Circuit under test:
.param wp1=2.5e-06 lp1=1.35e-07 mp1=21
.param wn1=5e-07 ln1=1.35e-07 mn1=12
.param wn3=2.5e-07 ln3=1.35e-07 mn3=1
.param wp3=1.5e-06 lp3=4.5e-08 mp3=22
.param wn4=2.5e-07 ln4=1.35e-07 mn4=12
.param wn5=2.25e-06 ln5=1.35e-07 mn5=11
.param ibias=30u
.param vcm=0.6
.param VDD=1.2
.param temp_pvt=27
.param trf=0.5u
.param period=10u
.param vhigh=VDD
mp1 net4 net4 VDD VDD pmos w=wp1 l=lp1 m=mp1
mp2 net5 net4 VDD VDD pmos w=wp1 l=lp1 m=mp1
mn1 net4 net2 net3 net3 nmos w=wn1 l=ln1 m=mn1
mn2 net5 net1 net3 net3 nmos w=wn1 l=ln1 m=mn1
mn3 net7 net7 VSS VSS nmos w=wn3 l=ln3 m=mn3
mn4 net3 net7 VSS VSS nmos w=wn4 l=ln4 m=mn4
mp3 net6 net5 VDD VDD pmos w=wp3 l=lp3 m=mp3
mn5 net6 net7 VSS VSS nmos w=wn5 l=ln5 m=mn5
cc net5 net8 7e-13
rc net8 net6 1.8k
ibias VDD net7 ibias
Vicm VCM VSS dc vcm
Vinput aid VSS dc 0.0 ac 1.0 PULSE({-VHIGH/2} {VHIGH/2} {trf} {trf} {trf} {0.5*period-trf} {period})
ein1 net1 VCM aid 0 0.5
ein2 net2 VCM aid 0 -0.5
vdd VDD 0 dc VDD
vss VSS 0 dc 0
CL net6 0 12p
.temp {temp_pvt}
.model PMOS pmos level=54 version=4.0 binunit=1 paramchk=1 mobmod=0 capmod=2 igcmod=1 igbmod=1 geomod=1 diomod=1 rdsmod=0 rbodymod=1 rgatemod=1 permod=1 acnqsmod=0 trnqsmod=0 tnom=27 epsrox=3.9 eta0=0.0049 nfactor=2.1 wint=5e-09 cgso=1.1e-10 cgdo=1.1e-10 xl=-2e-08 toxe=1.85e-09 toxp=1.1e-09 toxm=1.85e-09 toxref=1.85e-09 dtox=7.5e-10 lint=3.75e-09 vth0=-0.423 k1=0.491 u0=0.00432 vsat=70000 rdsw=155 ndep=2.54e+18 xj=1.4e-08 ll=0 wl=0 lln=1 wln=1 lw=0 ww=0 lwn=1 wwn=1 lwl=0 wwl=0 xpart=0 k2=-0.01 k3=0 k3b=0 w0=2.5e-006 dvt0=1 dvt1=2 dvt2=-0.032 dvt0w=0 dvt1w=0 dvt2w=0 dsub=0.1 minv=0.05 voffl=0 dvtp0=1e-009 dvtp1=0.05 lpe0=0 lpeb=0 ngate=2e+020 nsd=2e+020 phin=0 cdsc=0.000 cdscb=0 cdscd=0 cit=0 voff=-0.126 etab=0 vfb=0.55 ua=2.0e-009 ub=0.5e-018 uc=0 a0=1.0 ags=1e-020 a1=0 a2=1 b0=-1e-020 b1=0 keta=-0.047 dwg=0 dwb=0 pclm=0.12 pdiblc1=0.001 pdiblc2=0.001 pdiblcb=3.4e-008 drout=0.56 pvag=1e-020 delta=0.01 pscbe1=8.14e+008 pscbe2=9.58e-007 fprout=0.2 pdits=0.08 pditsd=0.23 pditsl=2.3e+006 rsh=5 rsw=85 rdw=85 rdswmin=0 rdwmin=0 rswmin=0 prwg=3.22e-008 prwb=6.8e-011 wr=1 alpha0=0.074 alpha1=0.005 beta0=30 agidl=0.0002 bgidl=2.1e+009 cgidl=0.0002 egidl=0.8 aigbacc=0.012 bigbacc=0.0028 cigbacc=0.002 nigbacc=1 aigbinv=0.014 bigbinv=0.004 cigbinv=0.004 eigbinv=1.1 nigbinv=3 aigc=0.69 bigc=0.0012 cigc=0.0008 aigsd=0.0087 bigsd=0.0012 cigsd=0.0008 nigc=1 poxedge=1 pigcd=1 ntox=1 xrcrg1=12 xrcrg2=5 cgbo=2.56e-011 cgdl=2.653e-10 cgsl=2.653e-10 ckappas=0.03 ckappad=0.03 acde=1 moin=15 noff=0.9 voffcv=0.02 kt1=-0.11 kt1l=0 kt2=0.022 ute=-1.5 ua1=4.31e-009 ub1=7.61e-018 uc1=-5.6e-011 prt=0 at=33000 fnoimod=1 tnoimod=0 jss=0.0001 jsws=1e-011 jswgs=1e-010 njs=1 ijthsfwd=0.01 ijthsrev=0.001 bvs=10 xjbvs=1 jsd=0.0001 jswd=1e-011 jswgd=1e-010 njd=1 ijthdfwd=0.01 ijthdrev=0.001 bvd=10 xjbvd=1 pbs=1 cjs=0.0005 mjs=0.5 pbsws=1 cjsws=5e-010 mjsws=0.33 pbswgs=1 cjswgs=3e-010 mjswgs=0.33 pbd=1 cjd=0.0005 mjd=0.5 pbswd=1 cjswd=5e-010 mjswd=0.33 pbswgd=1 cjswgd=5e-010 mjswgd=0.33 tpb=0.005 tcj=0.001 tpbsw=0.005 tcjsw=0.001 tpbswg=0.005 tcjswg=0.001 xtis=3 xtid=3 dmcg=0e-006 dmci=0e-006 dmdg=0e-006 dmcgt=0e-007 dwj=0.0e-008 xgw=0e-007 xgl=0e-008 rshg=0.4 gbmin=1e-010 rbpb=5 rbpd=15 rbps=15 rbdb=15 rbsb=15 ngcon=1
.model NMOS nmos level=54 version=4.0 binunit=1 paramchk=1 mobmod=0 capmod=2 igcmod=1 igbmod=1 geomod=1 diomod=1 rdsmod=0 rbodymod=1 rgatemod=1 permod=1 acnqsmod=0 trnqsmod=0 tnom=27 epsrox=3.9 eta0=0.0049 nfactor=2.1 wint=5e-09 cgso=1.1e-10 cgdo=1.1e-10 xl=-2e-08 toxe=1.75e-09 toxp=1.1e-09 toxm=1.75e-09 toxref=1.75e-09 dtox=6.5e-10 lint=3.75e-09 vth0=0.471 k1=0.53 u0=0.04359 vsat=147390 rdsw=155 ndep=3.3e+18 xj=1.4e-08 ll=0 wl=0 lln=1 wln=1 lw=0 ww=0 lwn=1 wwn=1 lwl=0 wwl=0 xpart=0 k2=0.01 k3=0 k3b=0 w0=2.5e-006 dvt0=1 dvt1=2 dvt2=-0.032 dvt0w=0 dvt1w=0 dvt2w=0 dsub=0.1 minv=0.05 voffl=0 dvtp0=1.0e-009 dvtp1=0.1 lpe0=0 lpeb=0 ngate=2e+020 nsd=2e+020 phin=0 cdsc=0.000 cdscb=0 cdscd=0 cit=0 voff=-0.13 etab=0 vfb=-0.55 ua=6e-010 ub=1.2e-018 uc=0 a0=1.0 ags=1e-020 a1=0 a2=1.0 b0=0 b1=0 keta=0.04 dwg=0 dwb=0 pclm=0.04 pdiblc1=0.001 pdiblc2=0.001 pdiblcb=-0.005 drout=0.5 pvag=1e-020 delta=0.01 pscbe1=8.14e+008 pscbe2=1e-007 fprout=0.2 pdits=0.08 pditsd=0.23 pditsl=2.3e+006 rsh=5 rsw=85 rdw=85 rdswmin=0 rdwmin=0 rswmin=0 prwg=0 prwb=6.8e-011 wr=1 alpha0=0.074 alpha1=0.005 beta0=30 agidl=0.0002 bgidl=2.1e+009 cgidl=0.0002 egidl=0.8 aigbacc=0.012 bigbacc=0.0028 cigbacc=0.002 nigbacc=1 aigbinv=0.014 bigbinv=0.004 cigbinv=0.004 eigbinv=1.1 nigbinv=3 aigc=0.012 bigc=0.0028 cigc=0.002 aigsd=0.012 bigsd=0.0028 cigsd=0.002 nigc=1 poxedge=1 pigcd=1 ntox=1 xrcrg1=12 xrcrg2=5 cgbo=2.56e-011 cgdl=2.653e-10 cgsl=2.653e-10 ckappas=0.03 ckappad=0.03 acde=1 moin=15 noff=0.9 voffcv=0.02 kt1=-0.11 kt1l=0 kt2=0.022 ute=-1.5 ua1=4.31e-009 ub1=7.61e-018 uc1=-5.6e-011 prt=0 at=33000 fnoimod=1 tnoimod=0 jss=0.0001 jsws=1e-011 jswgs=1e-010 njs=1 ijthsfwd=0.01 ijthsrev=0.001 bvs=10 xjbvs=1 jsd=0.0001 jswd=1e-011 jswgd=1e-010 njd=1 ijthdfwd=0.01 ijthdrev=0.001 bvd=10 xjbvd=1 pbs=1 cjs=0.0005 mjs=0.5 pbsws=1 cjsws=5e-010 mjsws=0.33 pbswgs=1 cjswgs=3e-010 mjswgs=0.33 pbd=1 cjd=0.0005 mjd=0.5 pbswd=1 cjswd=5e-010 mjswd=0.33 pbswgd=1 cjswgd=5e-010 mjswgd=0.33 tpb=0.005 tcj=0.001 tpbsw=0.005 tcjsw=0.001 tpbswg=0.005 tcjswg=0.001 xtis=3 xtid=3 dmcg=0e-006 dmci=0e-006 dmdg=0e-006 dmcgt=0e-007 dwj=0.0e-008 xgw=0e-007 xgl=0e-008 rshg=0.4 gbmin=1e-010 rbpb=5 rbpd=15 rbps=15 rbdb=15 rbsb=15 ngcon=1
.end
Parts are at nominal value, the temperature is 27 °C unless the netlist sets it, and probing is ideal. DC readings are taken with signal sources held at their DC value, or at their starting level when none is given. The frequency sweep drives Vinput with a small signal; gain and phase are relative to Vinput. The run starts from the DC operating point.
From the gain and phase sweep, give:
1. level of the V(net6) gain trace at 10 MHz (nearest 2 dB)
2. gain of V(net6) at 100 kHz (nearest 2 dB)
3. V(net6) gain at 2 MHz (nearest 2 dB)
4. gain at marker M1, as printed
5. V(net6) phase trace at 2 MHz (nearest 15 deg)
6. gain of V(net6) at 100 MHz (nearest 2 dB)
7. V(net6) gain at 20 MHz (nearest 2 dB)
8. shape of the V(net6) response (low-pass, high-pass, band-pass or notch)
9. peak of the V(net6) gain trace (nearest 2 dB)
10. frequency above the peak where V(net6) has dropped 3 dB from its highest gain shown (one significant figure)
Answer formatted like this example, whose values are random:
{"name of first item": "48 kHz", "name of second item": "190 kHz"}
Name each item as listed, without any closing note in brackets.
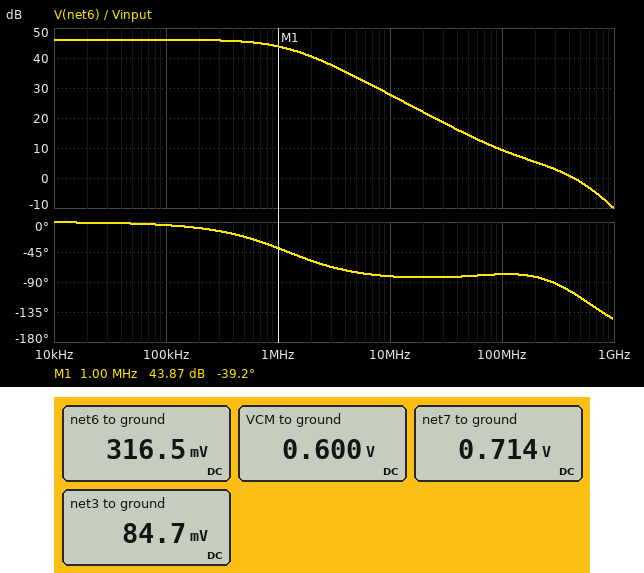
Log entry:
{"level of the V(net6) gain trace at 10 MHz": "28 dB", "gain of V(net6) at 100 kHz": "46 dB", "V(net6) gain at 2 MHz": "40 dB", "gain at marker M1, as printed": "43.87 dB", "V(net6) phase trace at 2 MHz": "-60 deg", "gain of V(net6) at 100 MHz": "10 dB", "V(net6) gain at 20 MHz": "22 dB", "shape of the V(net6) response": "low-pass", "peak of the V(net6) gain trace": "46 dB", "frequency above the peak where V(net6) has dropped 3 dB from its highest gain shown": "1 MHz"}
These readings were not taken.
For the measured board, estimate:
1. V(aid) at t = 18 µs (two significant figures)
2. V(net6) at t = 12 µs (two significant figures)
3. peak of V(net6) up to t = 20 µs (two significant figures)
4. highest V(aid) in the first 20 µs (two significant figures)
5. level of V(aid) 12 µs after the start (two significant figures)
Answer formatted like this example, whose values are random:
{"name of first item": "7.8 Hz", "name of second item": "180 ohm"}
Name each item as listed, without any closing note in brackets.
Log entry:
{"V(aid) at t = 18 µs": "-600 mV", "V(net6) at t = 12 µs": "1.1 V", "peak of V(net6) up to t = 20 µs": "1.1 V", "highest V(aid) in the first 20 µs": "600 mV", "level of V(aid) 12 µs after the start": "600 mV"}
